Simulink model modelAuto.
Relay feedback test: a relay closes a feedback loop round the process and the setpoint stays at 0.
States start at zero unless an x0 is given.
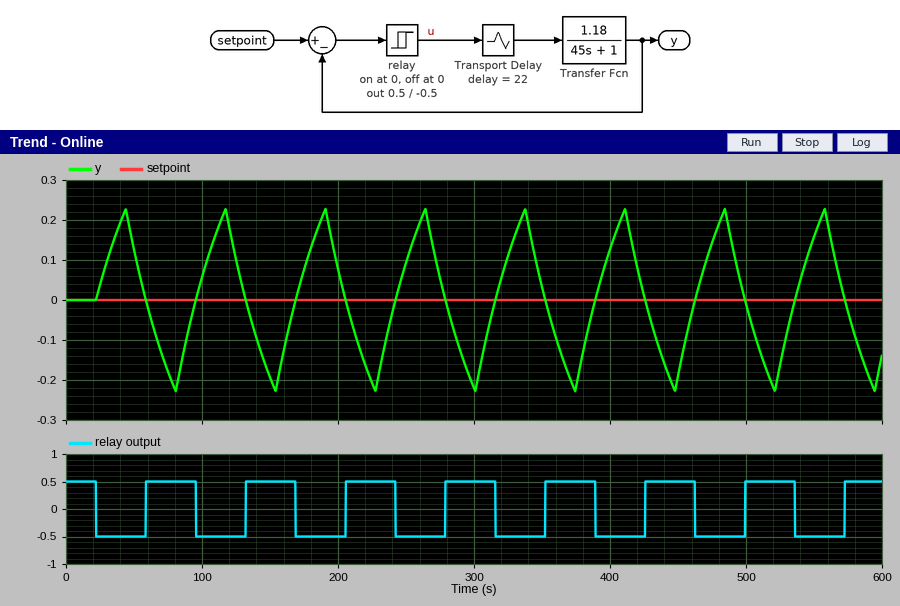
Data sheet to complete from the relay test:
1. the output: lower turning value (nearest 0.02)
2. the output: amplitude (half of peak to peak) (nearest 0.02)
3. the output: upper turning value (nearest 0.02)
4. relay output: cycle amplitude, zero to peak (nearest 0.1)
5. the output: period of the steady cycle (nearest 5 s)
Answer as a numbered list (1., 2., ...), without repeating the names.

1. -0.22
2. 0.22
3. 0.22
4. 0.5
5. 75 s
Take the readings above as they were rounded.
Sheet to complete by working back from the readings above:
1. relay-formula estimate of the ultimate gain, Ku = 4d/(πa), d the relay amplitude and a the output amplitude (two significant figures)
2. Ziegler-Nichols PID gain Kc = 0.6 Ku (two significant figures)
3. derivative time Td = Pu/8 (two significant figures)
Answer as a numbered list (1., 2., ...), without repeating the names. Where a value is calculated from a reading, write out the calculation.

1. 4 × 0.5 / (π × 0.22) = 2.9
2. 0.6 × 2.9 = 1.7
3. 75 / 8 = 9.4 s
